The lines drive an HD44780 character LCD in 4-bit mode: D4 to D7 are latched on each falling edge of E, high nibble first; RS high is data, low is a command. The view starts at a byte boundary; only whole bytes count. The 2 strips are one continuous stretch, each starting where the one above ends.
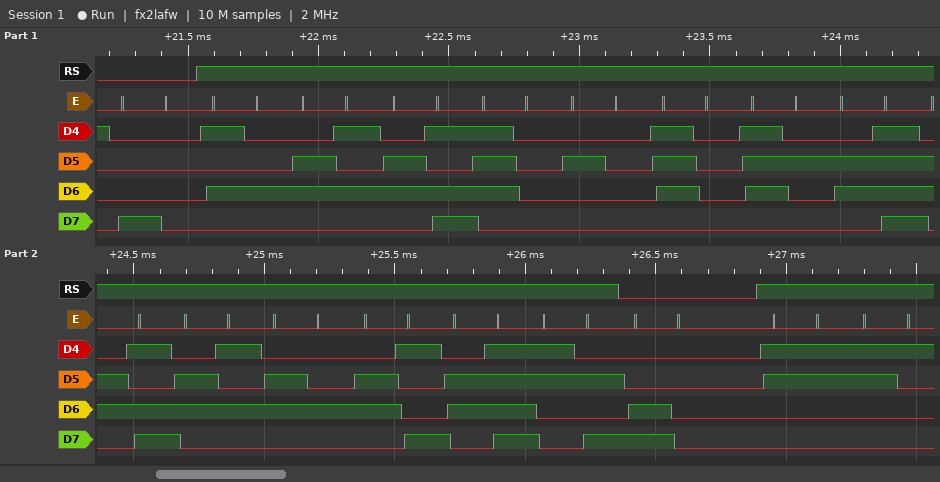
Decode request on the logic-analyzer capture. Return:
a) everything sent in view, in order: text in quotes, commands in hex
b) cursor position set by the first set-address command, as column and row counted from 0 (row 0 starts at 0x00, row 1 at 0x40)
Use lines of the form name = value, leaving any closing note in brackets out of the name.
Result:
everything sent in view, in order: text in quotes, commands in hex = 0x80 "Temp promedio:" 0xC0 "31"
cursor position set by the first set-address command, as column and row counted from 0 = column 0, row 0
